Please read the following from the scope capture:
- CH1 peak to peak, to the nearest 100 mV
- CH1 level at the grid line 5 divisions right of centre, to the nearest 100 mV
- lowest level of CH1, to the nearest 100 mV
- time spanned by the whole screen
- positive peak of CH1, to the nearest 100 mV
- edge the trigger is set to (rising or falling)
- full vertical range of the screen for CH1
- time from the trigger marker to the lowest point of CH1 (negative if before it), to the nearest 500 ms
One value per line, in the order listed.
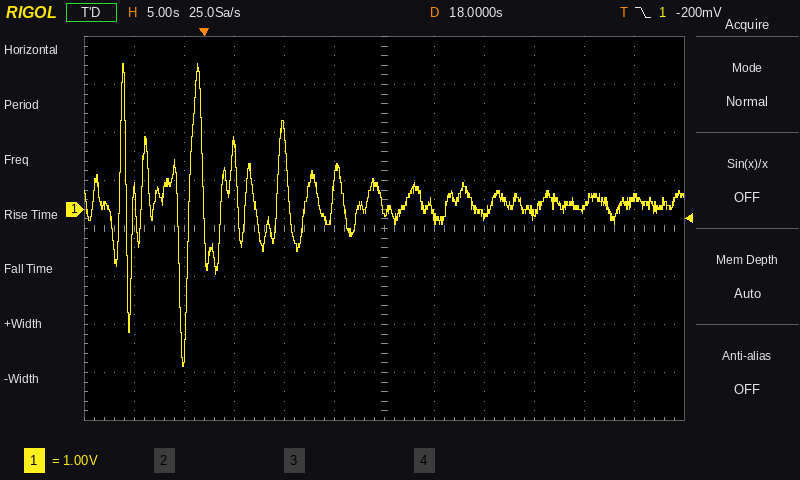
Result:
6.3 V
200 mV
-3.3 V
60 s
3.0 V
falling
8 V
-2.0 s
